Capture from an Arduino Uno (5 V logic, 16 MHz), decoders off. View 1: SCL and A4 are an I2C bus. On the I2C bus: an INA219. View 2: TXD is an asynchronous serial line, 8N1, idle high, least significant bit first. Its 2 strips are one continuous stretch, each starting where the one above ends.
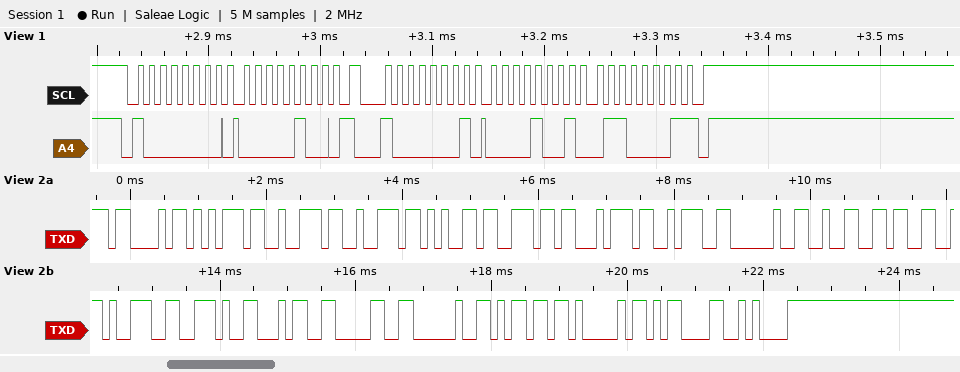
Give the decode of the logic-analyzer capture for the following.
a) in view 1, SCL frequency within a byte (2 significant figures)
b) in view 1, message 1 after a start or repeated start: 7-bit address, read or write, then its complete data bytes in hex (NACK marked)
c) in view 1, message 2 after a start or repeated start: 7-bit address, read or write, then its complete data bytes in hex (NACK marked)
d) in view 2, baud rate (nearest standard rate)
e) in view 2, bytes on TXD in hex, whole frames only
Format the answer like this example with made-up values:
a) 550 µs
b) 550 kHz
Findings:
a) 100 kHz
b) 0x40 write: 04
c) 0x40 read: 09 61 NACK
d) 9600 baud
e) 43 75 72 72 65 6E 74 3A 20 32 33 39 2E 34 30 20 6D 41 0D 0A
